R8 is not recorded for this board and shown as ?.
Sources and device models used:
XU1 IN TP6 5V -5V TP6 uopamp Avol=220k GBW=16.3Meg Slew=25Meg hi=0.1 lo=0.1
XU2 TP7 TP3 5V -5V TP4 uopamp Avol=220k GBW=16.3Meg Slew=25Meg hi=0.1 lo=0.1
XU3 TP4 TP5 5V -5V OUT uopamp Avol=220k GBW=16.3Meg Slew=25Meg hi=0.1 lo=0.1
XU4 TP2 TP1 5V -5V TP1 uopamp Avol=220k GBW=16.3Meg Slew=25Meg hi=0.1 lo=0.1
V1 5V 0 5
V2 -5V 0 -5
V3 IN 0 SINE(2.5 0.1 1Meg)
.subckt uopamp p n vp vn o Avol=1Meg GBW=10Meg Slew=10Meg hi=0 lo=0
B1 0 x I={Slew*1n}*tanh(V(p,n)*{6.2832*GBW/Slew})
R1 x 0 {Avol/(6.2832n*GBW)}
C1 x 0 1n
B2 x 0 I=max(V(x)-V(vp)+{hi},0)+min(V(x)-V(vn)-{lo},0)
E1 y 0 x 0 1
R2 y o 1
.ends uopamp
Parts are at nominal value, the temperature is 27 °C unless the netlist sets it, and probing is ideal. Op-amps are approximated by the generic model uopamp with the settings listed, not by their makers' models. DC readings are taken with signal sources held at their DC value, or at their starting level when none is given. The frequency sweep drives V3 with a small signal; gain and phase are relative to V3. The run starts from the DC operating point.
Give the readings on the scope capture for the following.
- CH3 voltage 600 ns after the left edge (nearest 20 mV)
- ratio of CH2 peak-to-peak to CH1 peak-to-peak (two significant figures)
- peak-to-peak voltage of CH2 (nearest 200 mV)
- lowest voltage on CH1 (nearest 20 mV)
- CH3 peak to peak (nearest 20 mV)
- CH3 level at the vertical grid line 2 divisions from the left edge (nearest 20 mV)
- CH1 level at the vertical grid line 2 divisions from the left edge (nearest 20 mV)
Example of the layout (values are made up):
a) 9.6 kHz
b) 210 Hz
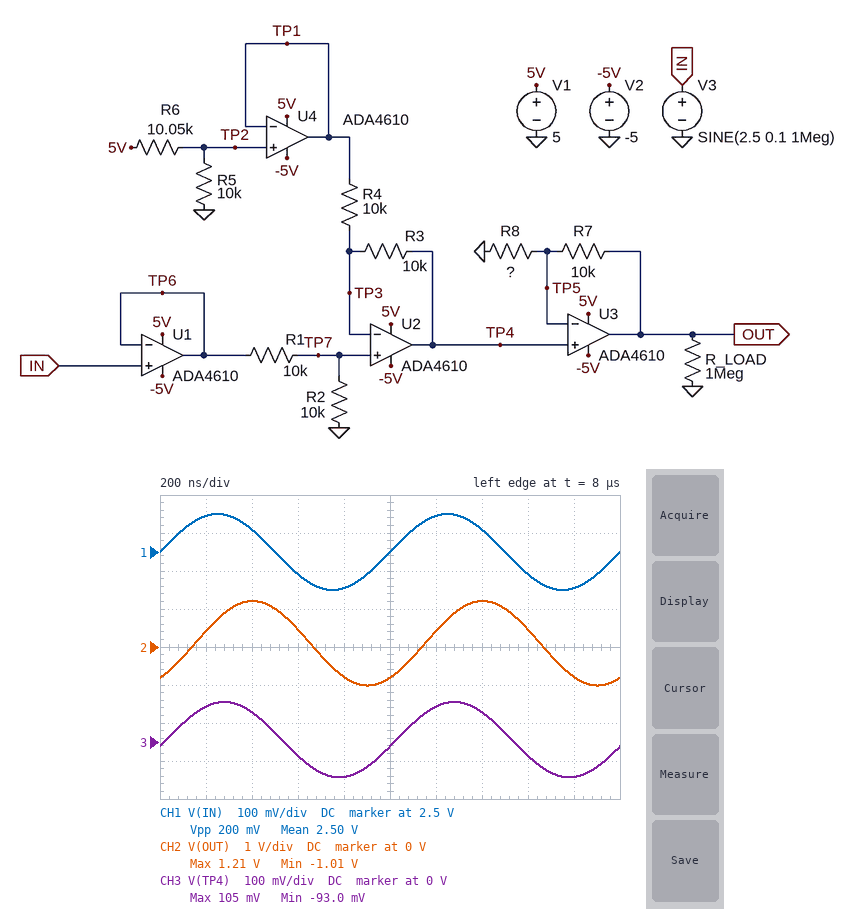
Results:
a) -40 mV
b) 11
c) 2.2 V
d) 2.40 V
e) 200 mV
f) 80 mV
g) 2.56 V
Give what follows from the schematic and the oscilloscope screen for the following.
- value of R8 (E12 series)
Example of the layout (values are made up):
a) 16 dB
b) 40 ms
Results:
a) 680 Ω
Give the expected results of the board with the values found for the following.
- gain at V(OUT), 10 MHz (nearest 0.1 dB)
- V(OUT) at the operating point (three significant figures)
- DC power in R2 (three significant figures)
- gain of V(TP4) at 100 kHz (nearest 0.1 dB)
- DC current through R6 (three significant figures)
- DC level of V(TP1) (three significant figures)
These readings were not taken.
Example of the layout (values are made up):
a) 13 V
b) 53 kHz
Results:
a) -1.2 dB
b) 97.9 mV
c) 156 µW
d) 0 dB
e) 249 µA
f) 2.49 V
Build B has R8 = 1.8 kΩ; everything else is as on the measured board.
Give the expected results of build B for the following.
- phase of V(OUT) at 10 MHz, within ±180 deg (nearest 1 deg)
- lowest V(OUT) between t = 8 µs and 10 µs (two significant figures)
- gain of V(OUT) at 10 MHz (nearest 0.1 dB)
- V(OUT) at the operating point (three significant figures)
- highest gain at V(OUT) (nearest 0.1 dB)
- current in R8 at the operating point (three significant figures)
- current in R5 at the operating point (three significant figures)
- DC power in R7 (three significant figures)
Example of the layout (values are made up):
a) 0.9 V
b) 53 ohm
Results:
a) -158 deg
b) -560 mV
c) -1.4 dB
d) 40.9 mV
e) 16.3 dB
f) 3.46 µA
g) 249 µA
h) 120 nW
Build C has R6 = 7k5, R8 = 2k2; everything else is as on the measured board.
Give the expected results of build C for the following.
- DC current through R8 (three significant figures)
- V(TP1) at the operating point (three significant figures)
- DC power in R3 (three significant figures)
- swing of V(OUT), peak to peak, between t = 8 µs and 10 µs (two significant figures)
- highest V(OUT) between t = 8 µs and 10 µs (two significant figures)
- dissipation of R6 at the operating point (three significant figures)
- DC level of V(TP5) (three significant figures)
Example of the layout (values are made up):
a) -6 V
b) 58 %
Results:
a) 162 µA
b) 2.86 V
c) 258 µW
d) 1.0 V
e) -1.5 V
f) 612 µW
g) -357 mV
